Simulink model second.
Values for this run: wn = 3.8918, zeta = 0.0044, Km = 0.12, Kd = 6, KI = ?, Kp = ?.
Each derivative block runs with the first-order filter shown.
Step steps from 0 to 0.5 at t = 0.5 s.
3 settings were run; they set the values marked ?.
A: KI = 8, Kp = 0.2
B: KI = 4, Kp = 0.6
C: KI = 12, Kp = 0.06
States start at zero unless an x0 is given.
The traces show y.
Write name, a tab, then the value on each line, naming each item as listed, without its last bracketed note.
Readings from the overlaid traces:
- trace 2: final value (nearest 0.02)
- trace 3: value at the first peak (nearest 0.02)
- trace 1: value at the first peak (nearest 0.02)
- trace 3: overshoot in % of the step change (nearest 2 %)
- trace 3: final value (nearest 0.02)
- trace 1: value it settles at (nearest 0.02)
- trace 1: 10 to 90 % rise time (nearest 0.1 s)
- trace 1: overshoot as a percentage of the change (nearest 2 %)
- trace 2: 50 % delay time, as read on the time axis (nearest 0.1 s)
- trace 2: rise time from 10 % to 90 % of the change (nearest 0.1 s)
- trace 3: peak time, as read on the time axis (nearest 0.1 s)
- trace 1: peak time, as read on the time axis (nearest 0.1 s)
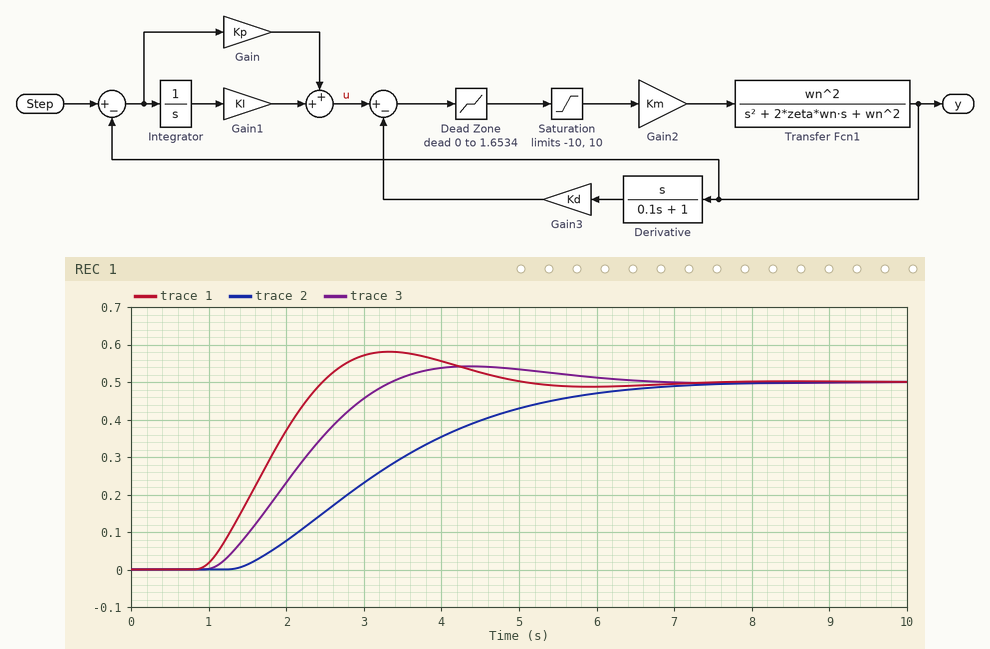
trace 2: final value	0.50
trace 3: value at the first peak	0.54
trace 1: value at the first peak	0.58
trace 3: overshoot in % of the step change	8 %
trace 3: final value	0.50
trace 1: value it settles at	0.50
trace 1: 10 to 90 % rise time	1.1 s
trace 1: overshoot as a percentage of the change	16 %
trace 2: 50 % delay time, as read on the time axis	3.1 s
trace 2: rise time from 10 % to 90 % of the change	3.6 s
trace 3: peak time, as read on the time axis	4.4 s
trace 1: peak time, as read on the time axis	3.3 s
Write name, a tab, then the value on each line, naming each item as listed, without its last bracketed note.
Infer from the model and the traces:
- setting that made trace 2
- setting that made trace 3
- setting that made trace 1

setting that made trace 2	B
setting that made trace 3	A
setting that made trace 1	C
